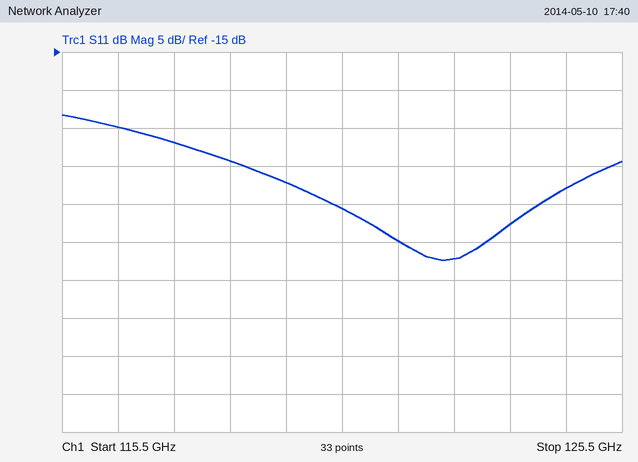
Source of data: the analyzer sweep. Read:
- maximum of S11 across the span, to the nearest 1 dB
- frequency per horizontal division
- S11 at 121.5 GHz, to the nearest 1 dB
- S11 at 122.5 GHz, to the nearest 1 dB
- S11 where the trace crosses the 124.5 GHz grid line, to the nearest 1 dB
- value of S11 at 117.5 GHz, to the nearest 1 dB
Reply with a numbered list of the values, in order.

1. -23 dB
2. 1 GHz
3. -40 dB
4. -42 dB
5. -33 dB
6. -27 dB
